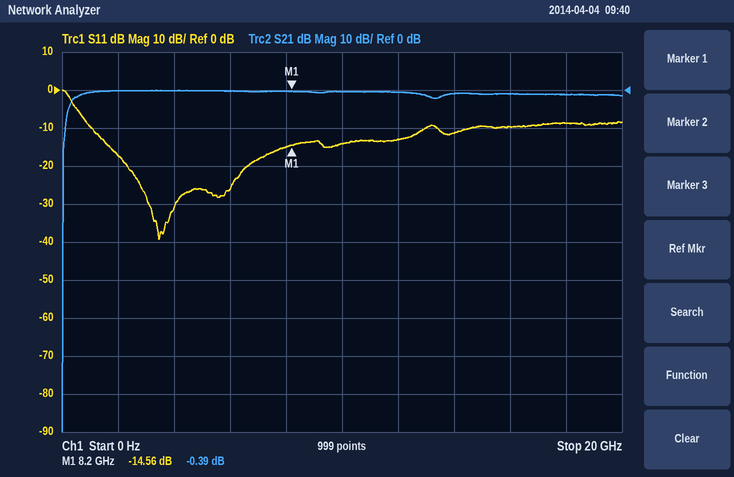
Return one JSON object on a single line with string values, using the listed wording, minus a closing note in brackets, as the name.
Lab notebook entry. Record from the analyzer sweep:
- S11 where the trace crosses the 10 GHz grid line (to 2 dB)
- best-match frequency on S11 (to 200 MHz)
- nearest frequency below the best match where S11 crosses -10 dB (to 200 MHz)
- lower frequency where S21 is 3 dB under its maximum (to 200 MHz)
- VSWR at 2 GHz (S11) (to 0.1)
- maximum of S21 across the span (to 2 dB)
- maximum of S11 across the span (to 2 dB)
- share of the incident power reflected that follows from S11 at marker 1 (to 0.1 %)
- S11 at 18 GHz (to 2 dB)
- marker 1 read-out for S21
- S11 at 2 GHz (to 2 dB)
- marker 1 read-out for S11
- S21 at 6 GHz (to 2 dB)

{"S11 where the trace crosses the 10 GHz grid line": "-14 dB", "best-match frequency on S11": "3.4 GHz", "nearest frequency below the best match where S11 crosses -10 dB": "1.0 GHz", "lower frequency where S21 is 3 dB under its maximum": "400 MHz", "VSWR at 2 GHz (S11)": "1.3", "maximum of S21 across the span": "0 dB", "maximum of S11 across the span": "0 dB", "share of the incident power reflected that follows from S11 at marker 1": "3.5 %", "S11 at 18 GHz": "-8 dB", "marker 1 read-out for S21": "-0.39 dB", "S11 at 2 GHz": "-18 dB", "marker 1 read-out for S11": "-14.56 dB", "S21 at 6 GHz": "0 dB"}
